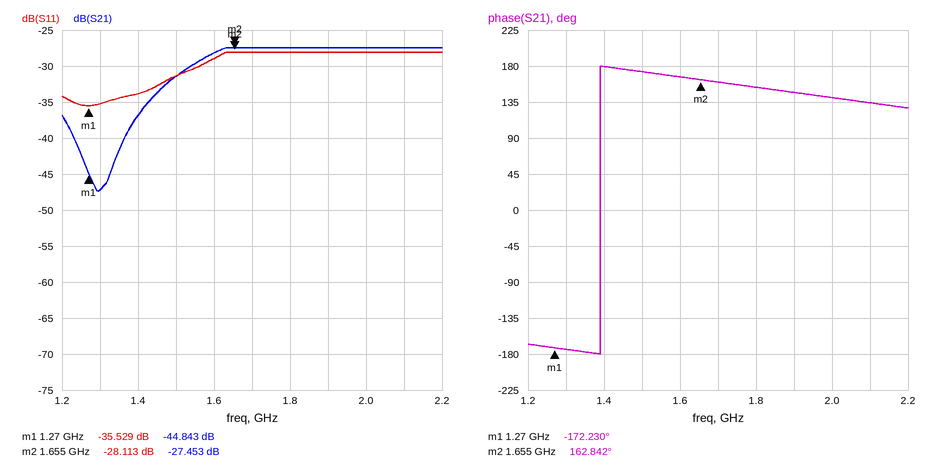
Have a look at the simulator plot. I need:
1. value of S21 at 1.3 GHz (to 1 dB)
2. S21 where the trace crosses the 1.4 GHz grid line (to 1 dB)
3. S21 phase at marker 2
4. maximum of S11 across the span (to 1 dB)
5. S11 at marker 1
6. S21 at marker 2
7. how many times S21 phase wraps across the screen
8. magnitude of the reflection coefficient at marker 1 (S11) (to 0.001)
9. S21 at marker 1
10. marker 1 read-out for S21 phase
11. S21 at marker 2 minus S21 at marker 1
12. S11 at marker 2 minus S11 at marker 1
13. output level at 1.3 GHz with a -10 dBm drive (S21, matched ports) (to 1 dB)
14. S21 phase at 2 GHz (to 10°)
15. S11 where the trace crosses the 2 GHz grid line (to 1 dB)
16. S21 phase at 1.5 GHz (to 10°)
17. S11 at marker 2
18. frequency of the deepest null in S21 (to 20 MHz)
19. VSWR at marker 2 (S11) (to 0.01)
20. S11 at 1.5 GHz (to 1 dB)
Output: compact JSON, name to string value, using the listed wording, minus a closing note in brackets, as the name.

{"value of S21 at 1.3 GHz": "-47 dB", "S21 where the trace crosses the 1.4 GHz grid line": "-37 dB", "S21 phase at marker 2": "162.842°", "maximum of S11 across the span": "-28 dB", "S11 at marker 1": "-35.529 dB", "S21 at marker 2": "-27.453 dB", "how many times S21 phase wraps across the screen": "1", "magnitude of the reflection coefficient at marker 1 (S11)": "0.017", "S21 at marker 1": "-44.843 dB", "marker 1 read-out for S21 phase": "-172.230°", "S21 at marker 2 minus S21 at marker 1": "17.390 dB", "S11 at marker 2 minus S11 at marker 1": "7.416 dB", "output level at 1.3 GHz with a -10 dBm drive (S21, matched ports)": "-57 dBm", "S21 phase at 2 GHz": "140°", "S11 where the trace crosses the 2 GHz grid line": "-28 dB", "S21 phase at 1.5 GHz": "170°", "S11 at marker 2": "-28.113 dB", "frequency of the deepest null in S21": "1.30 GHz", "VSWR at marker 2 (S11)": "1.08", "S11 at 1.5 GHz": "-31 dB"}
